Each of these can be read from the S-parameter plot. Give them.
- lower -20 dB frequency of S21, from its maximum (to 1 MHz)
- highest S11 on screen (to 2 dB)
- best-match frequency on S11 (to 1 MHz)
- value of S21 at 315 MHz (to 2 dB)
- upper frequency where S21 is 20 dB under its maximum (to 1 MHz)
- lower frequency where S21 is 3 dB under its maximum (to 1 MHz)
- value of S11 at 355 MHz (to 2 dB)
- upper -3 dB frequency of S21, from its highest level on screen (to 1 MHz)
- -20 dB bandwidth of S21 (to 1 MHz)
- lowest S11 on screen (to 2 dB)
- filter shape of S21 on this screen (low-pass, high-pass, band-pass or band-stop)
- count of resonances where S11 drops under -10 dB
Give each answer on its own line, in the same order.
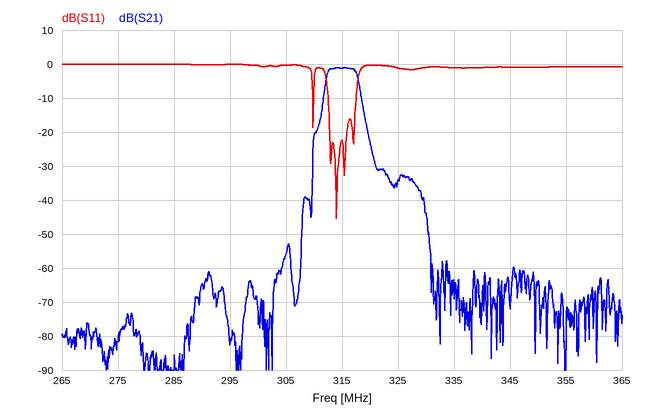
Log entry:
310 MHz
0 dB
314 MHz
-2 dB
320 MHz
312 MHz
0 dB
318 MHz
10 MHz
-46 dB
band-pass
5
